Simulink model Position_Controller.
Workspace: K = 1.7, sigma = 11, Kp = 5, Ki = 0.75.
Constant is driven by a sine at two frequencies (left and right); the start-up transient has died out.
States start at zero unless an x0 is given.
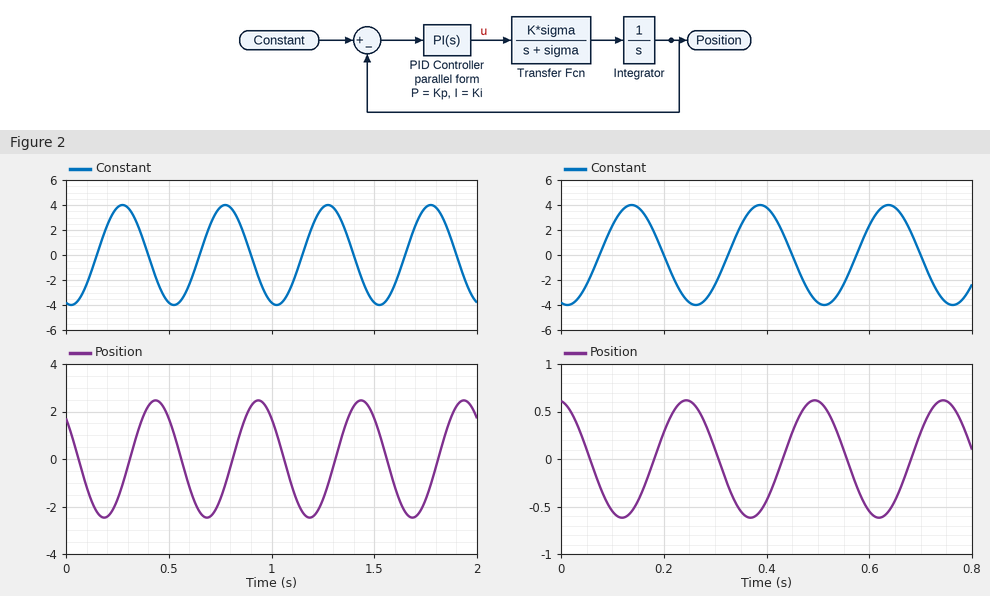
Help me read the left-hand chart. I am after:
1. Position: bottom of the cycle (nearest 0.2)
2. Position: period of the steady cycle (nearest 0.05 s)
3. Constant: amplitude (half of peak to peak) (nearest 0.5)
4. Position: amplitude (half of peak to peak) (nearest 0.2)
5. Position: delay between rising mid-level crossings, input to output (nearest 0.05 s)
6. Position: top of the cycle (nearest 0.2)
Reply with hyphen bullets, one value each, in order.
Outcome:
- -2.4
- 0.50 s
- 4.0
- 2.4
- 0.15 s
- 2.4
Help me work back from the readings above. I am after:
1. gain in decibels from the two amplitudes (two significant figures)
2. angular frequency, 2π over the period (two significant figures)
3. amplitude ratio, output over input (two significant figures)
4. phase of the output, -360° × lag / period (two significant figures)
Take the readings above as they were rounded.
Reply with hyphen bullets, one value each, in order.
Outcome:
- -4.4 dB
- 13 rad/s
- 0.60
- -110°
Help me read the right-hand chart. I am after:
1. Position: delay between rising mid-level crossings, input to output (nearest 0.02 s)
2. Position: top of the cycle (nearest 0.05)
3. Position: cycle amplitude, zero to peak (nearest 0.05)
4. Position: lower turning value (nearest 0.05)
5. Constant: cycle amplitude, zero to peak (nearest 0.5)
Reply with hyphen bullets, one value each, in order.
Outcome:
- 0.10 s
- 0.60
- 0.60
- -0.60
- 4.0
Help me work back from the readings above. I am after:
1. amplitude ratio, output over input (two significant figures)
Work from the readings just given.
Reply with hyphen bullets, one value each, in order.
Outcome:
- 0.15
